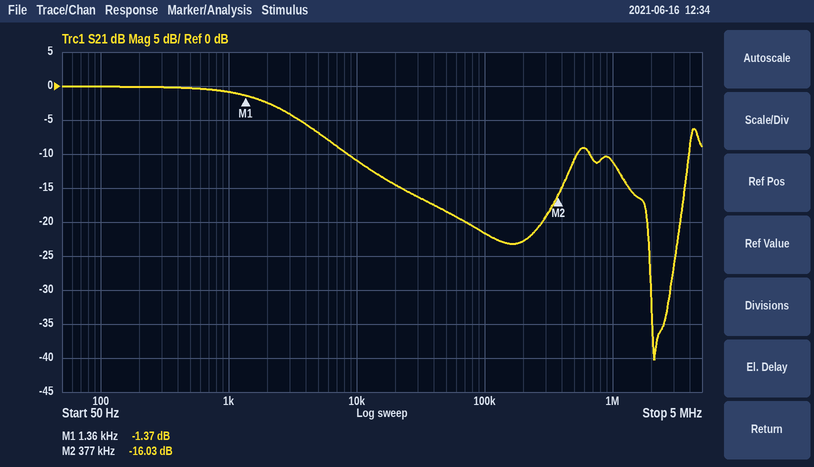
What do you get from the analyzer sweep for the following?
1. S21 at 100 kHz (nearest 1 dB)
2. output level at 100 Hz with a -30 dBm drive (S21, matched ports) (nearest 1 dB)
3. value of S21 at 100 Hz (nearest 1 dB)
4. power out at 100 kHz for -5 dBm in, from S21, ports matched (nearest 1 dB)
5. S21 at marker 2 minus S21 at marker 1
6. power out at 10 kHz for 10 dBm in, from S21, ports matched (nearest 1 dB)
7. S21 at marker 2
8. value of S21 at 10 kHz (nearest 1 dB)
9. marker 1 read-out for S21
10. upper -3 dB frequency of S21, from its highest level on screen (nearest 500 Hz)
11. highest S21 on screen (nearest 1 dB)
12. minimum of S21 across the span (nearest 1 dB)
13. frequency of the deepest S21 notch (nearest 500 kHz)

-22 dB
-30 dBm
0 dB
-27 dBm
-14.66 dB
-1 dBm
-16.03 dB
-11 dB
-1.37 dB
2.5 kHz
0 dB
-40 dB
2.0 MHz
